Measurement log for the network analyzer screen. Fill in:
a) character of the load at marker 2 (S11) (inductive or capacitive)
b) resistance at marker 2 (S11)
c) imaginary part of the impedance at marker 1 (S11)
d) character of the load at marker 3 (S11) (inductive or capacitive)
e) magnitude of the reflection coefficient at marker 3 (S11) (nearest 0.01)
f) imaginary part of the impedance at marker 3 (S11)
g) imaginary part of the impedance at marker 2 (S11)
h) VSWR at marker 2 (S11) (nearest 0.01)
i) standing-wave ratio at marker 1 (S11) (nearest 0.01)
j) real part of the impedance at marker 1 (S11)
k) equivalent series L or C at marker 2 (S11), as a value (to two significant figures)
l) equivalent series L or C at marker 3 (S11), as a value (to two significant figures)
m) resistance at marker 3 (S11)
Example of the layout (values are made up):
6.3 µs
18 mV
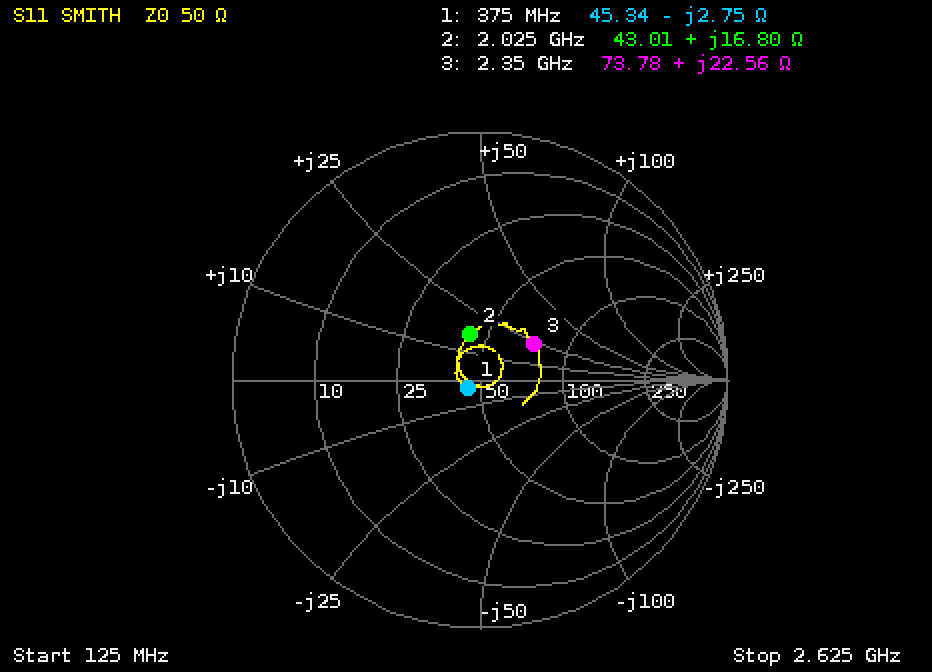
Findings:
inductive
43.01 Ω
-2.75 Ω
inductive
0.26
+22.56 Ω
+16.80 Ω
1.48
1.12
45.34 Ω
1.3 nH
1.5 nH
73.78 Ω
